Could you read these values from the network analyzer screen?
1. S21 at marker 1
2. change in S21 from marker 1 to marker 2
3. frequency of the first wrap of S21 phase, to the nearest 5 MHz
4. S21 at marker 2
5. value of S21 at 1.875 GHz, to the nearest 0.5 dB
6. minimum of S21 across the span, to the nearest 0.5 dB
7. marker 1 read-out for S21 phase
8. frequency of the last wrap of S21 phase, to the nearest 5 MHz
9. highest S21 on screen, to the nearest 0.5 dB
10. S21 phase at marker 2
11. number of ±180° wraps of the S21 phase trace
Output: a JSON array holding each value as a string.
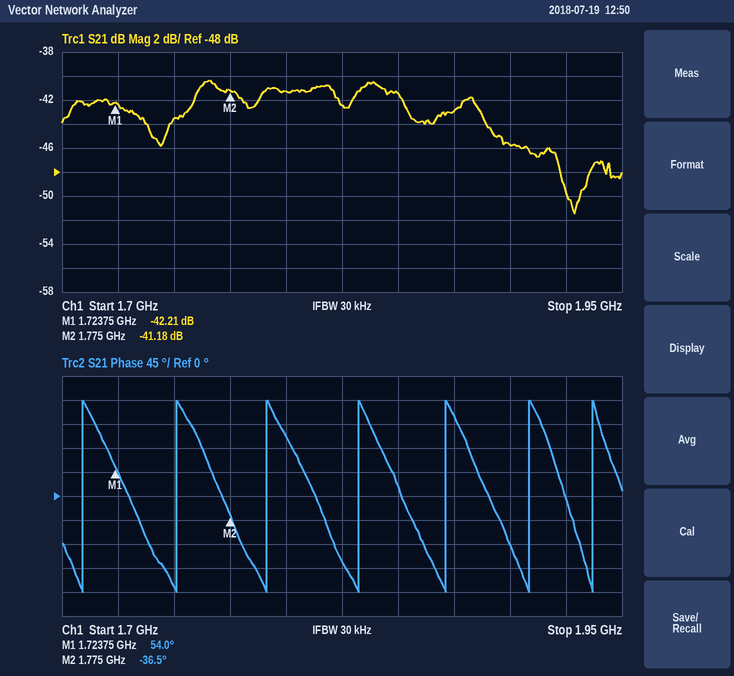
["-42.21 dB", "1.03 dB", "1.710 GHz", "-41.18 dB", "-43.0 dB", "-51.5 dB", "54.0°", "1.935 GHz", "-40.5 dB", "-36.5°", "7"]
